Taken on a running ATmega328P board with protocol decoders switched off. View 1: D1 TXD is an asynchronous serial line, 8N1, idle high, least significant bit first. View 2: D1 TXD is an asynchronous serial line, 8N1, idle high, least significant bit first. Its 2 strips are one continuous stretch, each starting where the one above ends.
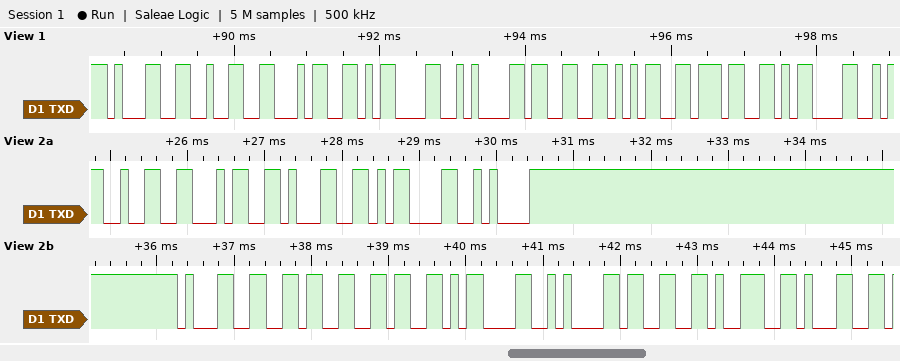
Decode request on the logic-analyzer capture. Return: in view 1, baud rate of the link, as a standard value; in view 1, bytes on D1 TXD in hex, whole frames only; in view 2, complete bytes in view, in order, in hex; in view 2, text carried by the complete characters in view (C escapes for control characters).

9600 baud
31 32 34 0D 0A 33 35 37 0D
32 34 31 0D 0A 31 36 36 0D 0A 33 39 31
"241\r\n166\r\n391"
